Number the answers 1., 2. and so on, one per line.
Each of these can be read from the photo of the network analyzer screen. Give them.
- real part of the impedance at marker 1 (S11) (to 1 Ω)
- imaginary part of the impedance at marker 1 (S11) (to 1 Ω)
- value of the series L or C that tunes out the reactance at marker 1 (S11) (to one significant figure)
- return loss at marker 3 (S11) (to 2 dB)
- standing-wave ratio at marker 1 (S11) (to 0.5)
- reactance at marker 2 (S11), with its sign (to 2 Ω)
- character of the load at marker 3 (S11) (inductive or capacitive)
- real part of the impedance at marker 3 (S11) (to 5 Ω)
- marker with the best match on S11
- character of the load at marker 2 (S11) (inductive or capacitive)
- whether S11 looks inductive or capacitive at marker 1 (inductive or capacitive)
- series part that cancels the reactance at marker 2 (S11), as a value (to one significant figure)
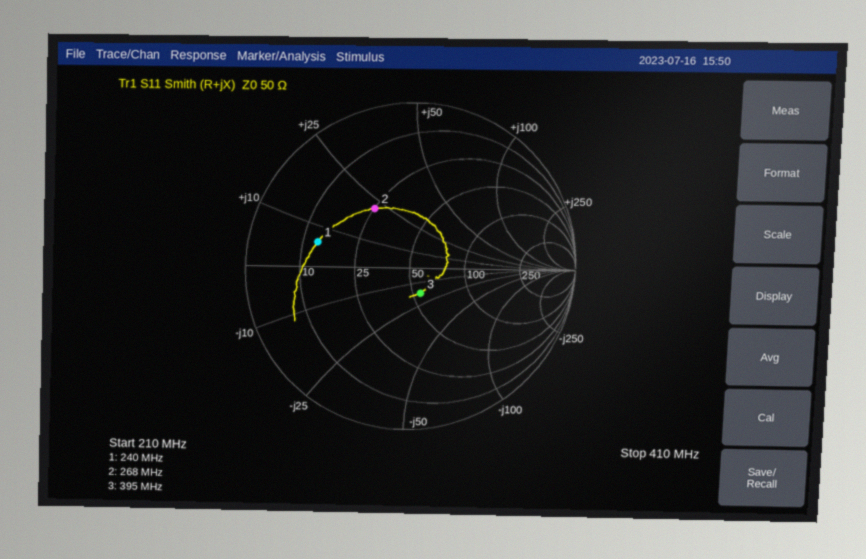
1. 13 Ω
2. +6 Ω
3. 100 pF
4. 16 dB
5. 4.0
6. +22 Ω
7. capacitive
8. 55 Ω
9. marker 3
10. inductive
11. inductive
12. 30 pF
